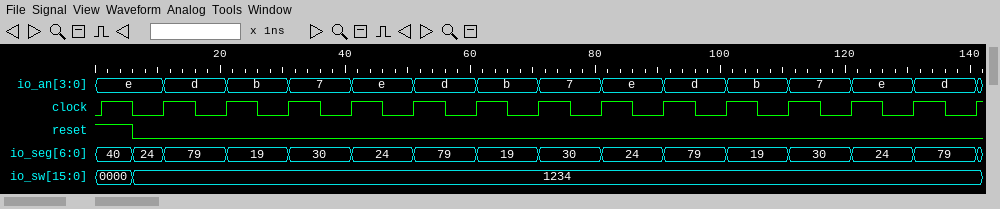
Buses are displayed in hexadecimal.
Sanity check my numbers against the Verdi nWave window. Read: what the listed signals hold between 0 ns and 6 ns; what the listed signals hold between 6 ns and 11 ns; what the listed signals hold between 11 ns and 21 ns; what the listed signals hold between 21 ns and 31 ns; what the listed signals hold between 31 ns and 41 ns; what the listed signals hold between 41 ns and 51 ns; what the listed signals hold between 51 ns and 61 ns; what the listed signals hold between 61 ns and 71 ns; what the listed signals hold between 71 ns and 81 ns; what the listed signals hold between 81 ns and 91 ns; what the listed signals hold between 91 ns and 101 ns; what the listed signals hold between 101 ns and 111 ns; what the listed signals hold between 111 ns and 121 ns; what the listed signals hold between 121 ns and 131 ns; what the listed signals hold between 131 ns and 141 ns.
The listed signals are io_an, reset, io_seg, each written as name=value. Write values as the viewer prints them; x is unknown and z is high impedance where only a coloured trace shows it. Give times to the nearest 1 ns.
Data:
io_an=e, reset=1, io_seg=40
io_an=e, reset=0, io_seg=24
io_an=d, reset=0, io_seg=79
io_an=b, reset=0, io_seg=19
io_an=7, reset=0, io_seg=30
io_an=e, reset=0, io_seg=24
io_an=d, reset=0, io_seg=79
io_an=b, reset=0, io_seg=19
io_an=7, reset=0, io_seg=30
io_an=e, reset=0, io_seg=24
io_an=d, reset=0, io_seg=79
io_an=b, reset=0, io_seg=19
io_an=7, reset=0, io_seg=30
io_an=e, reset=0, io_seg=24
io_an=d, reset=0, io_seg=79
